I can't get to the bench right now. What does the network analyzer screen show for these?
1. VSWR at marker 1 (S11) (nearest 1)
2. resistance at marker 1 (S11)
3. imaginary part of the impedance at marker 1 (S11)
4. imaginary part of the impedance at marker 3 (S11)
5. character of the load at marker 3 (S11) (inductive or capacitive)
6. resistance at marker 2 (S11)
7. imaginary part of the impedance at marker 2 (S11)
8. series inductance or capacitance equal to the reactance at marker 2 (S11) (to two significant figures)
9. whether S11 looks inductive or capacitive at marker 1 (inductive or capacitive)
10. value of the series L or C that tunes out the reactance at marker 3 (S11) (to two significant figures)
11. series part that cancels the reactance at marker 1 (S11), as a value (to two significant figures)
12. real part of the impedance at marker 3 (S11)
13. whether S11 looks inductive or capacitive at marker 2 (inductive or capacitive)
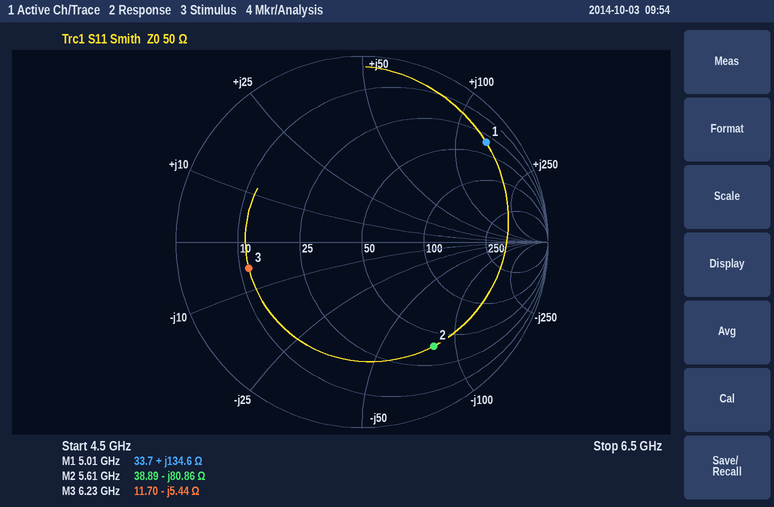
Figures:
13
33.7 Ω
+134.6 Ω
-5.44 Ω
capacitive
38.89 Ω
-80.86 Ω
350 fF
inductive
140 pH
240 fF
11.70 Ω
capacitive
